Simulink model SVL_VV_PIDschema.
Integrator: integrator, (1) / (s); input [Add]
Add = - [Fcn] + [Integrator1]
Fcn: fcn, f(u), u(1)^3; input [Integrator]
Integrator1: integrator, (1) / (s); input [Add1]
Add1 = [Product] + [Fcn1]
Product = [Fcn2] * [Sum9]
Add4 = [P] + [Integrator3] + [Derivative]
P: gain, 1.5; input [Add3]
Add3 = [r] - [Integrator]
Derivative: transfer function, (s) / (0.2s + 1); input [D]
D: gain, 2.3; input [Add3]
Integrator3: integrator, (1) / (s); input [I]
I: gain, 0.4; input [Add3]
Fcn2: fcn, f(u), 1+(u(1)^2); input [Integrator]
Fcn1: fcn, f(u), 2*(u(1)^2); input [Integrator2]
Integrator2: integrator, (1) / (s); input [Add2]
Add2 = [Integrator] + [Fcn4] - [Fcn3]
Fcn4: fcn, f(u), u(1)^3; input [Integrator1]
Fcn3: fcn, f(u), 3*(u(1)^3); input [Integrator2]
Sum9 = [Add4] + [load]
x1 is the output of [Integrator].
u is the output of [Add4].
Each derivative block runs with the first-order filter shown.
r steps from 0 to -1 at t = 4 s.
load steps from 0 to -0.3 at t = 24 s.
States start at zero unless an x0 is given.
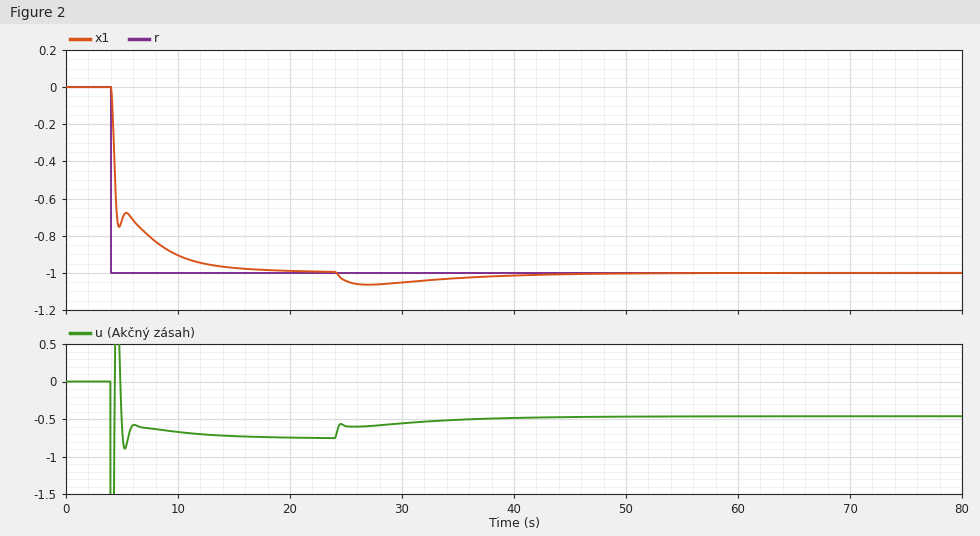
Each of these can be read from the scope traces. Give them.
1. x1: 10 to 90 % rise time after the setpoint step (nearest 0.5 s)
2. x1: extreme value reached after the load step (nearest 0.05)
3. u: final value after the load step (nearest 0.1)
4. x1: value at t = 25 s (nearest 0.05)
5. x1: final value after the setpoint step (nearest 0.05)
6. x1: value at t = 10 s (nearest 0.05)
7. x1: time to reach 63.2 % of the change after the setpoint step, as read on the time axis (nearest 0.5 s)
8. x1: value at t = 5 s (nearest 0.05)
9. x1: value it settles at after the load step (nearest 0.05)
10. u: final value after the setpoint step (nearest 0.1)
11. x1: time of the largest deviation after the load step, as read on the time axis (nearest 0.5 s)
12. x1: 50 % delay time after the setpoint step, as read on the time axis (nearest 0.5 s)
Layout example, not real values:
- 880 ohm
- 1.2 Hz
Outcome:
- 5.5 s
- -1.05
- -0.5
- -1.05
- -1.00
- -0.90
- 4.5 s
- -0.70
- -1.00
- -0.8
- 27.0 s
- 4.5 s
